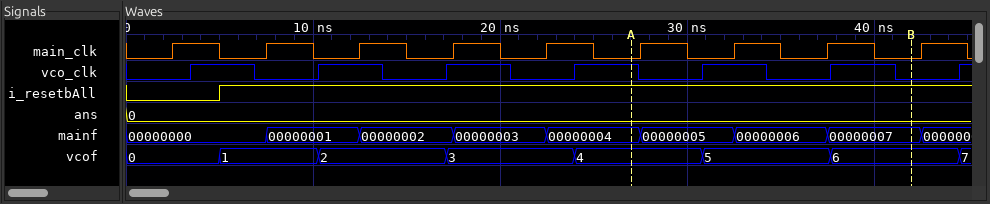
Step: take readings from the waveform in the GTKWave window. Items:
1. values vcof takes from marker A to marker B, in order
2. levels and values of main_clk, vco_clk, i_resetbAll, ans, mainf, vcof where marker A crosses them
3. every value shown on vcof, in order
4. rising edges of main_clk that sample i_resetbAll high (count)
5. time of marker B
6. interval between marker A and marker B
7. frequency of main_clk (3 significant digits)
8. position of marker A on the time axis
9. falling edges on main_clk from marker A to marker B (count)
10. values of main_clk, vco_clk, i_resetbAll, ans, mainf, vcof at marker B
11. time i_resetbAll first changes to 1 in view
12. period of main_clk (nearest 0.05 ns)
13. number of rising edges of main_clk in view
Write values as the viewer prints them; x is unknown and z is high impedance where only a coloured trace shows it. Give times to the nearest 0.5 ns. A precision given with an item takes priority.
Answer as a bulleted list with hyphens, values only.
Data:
- 4, 5, 6
- main_clk=0, vco_clk=1, i_resetbAll=1, ans=0, mainf=00000004, vcof=4
- 0, 1, 2, 3, 4, 5, 6, 7
- 8
- 42 ns
- 15 ns
- 200 MHz
- 27 ns
- 3
- main_clk=0, vco_clk=0, i_resetbAll=1, ans=0, mainf=00000007, vcof=6
- 5 ns
- 5 ns
- 9
